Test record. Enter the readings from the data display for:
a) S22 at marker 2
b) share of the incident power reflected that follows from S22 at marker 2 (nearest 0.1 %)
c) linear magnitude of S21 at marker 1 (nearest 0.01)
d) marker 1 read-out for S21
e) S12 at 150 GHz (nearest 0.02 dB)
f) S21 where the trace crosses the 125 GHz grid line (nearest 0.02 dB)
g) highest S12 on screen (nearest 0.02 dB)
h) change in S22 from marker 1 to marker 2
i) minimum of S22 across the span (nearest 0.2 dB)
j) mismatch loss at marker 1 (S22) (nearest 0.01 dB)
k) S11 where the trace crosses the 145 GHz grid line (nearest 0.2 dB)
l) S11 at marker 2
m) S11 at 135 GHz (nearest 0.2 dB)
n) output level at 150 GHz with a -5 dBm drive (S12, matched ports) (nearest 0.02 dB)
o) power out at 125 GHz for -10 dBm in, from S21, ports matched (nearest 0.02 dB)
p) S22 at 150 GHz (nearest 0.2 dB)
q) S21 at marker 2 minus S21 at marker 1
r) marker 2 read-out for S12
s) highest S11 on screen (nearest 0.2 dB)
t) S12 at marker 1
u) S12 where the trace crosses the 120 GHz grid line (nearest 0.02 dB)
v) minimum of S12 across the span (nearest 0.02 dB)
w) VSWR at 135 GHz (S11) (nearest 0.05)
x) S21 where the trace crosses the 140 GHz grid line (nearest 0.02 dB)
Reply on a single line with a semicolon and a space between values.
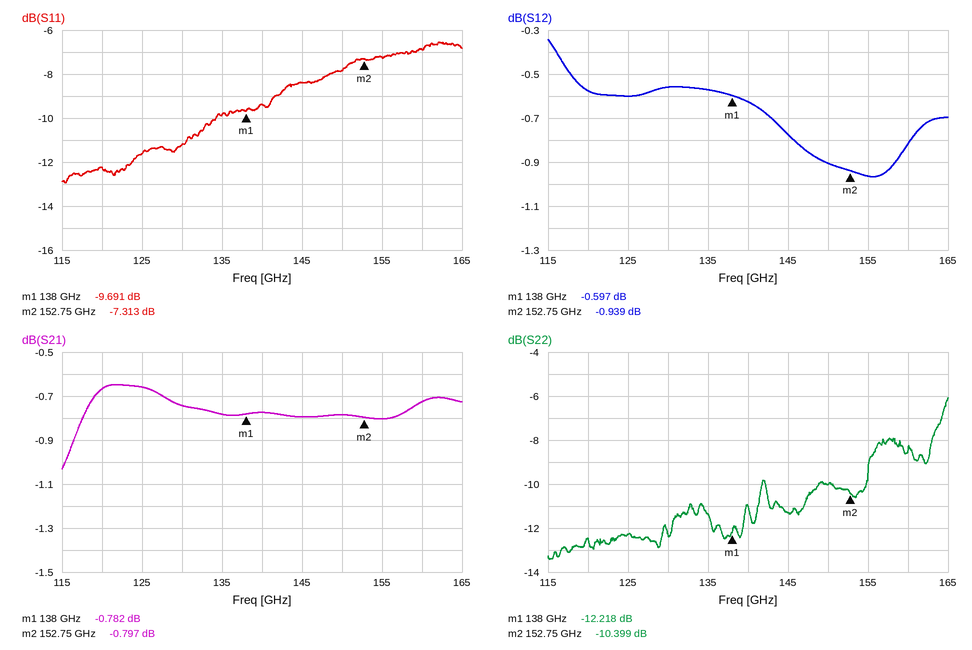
-10.399 dB; 9.1 %; 0.91; -0.782 dB; -0.90 dB; -0.66 dB; -0.34 dB; 1.819 dB; -13.4 dB; 0.27 dB; -8.4 dB; -7.313 dB; -9.8 dB; -5.90 dBm; -10.66 dBm; -10.0 dB; -0.015 dB; -0.939 dB; -6.6 dB; -0.597 dB; -0.58 dB; -0.96 dB; 1.95; -0.78 dB
